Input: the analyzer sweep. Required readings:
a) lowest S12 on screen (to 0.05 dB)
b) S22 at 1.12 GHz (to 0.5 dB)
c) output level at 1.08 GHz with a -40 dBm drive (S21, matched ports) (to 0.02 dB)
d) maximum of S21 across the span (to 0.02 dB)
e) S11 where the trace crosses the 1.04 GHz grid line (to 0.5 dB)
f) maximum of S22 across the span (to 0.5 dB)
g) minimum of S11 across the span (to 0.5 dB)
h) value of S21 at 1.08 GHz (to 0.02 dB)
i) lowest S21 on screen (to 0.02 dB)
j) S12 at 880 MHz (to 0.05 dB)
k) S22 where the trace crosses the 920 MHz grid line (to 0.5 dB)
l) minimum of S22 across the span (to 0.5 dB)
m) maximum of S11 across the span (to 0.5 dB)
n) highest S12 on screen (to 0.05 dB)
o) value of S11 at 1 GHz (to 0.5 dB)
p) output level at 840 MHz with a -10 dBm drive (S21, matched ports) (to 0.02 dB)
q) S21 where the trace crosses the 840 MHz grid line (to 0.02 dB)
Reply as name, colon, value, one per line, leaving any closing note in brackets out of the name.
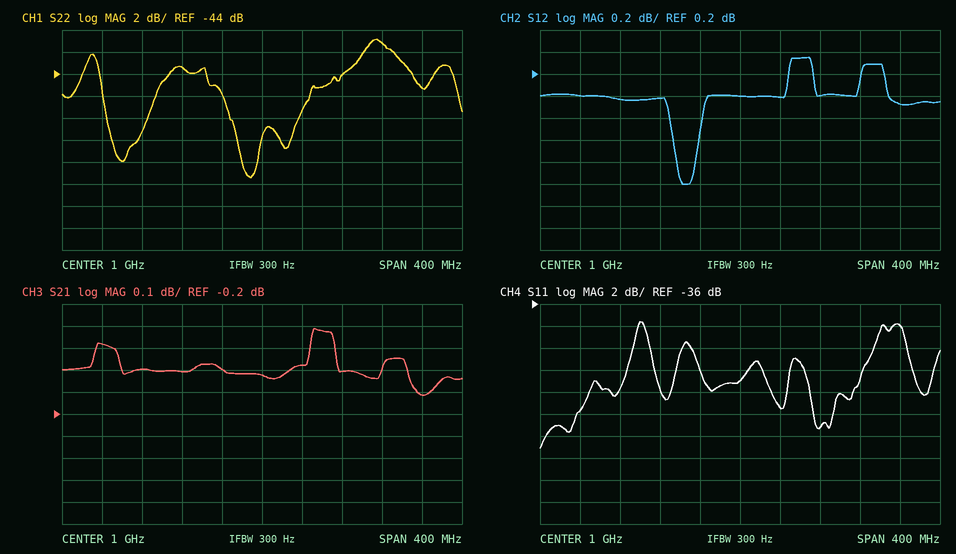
lowest S12 on screen: -0.80 dB
S22 at 1.12 GHz: -41.0 dB
output level at 1.08 GHz with a -40 dBm drive (S21, matched ports): -40.00 dBm
maximum of S21 across the span: 0.18 dB
S11 where the trace crosses the 1.04 GHz grid line: -45.5 dB
maximum of S22 across the span: -41.0 dB
minimum of S11 across the span: -49.0 dB
value of S21 at 1.08 GHz: 0.00 dB
lowest S21 on screen: -0.12 dB
S12 at 880 MHz: -0.05 dB
S22 where the trace crosses the 920 MHz grid line: -43.5 dB
minimum of S22 across the span: -53.5 dB
maximum of S11 across the span: -37.5 dB
highest S12 on screen: 0.35 dB
value of S11 at 1 GHz: -43.0 dB
output level at 840 MHz with a -10 dBm drive (S21, matched ports): -9.88 dBm
S21 where the trace crosses the 840 MHz grid line: 0.12 dB
